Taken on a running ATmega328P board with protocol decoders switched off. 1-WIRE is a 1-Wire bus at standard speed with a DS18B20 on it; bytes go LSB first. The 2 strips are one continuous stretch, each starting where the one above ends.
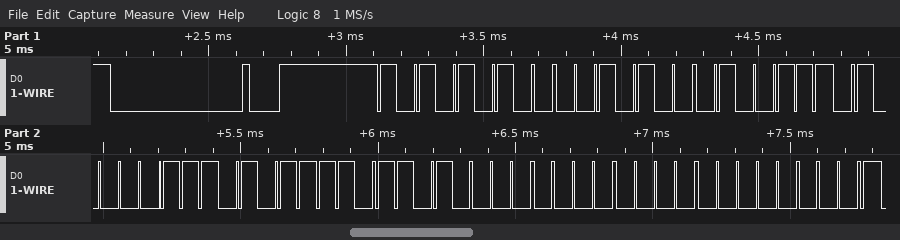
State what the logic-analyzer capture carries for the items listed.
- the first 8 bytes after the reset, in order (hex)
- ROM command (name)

55 28 72 E1 7A 0B 00 00
Match ROM
